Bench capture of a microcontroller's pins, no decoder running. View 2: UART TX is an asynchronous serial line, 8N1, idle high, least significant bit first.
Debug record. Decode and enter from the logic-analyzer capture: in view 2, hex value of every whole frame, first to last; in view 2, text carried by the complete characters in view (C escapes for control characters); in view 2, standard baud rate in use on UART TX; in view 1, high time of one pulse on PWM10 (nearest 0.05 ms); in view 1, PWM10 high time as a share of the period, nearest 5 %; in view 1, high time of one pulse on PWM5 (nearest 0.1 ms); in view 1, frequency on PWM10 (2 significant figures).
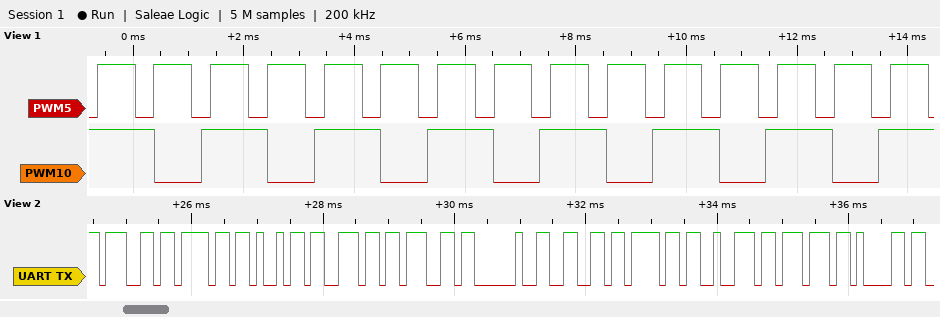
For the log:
0x67 0x6F 0x69 0x6E 0x67 0x20 0x66 0x6F 0x72 0x77 0x61
"going forwa"
9600 baud
1.20 ms
60 %
0.7 ms
490 Hz
